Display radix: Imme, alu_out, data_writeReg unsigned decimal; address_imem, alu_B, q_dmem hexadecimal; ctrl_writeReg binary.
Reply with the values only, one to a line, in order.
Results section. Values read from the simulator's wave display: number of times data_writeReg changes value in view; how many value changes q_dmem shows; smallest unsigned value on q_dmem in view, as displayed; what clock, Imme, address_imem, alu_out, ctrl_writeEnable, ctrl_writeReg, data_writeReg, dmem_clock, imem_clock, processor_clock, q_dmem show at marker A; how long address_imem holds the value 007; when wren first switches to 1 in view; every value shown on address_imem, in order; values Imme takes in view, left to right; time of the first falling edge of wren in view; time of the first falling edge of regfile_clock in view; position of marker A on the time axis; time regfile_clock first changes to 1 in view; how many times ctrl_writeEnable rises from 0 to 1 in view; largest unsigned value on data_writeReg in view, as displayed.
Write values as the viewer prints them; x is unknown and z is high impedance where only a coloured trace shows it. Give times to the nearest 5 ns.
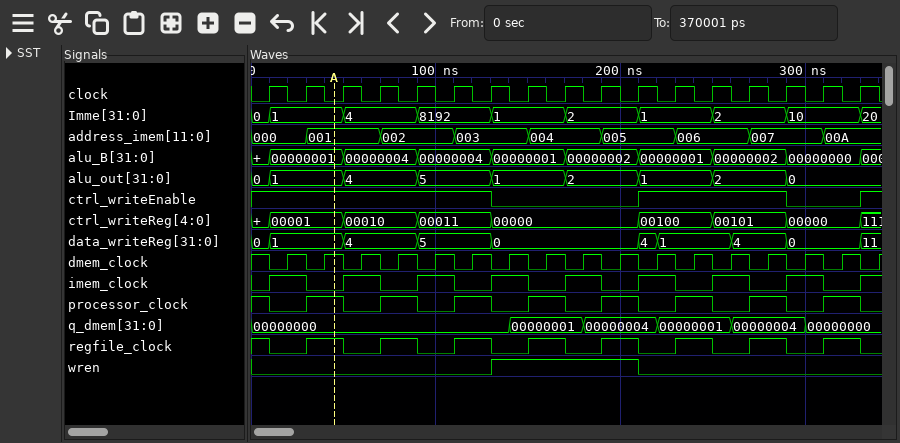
9
5
00000000
clock=0, Imme=1, address_imem=001, alu_out=1, ctrl_writeEnable=1, ctrl_writeReg=00001, data_writeReg=1, dmem_clock=1, imem_clock=0, processor_clock=1, q_dmem=00000000
40 ns
130 ns
000, 001, 002, 003, 004, 005, 006, 007, 00A
0, 1, 4, 8192, 1, 2, 1, 2, 10, 20
210 ns
10 ns
45 ns
30 ns
2
11
